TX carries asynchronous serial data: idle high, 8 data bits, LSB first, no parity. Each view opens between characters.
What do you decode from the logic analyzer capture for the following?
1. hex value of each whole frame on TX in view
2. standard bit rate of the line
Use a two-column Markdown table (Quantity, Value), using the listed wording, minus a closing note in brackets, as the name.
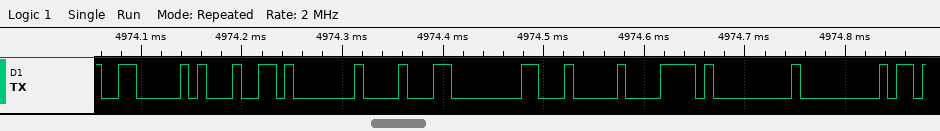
| Quantity | Value |
|---|---|
| hex value of each whole frame on TX in view | 06, 91, 01, 88, 80, 04, 78, 00, 00 |
| standard bit rate of the line | 115200 baud |
